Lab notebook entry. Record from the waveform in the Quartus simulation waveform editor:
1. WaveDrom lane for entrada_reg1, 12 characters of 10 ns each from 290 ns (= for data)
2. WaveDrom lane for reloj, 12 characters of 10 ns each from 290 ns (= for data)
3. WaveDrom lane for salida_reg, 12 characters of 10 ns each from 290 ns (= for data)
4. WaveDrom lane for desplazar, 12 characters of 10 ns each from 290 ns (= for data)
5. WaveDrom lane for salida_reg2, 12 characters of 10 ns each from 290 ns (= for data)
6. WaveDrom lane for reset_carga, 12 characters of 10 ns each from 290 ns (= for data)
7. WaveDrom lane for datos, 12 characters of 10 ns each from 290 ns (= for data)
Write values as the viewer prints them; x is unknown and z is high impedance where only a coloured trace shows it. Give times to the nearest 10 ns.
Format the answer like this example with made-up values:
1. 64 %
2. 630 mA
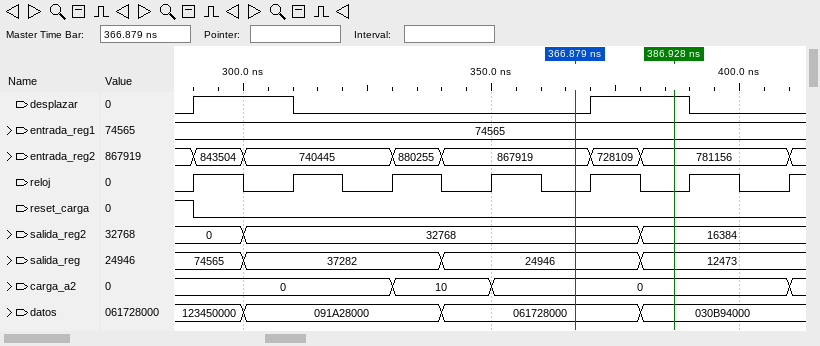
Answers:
1. {name: 'entrada_reg1', wave: '=...........', data: '74565'}
2. {name: 'reloj', wave: '101010101010'}
3. {name: 'salida_reg', wave: '==...=...=..', data: '74565 37282 24946 12473'}
4. {name: 'desplazar', wave: '1.0.....1.0.'}
5. {name: 'salida_reg2', wave: '==.......=..', data: '0 32768 16384'}
6. {name: 'reset_carga', wave: '0...........'}
7. {name: 'datos', wave: '==...=...=..', data: '123450000 091A28000 061728000 030B94000'}
